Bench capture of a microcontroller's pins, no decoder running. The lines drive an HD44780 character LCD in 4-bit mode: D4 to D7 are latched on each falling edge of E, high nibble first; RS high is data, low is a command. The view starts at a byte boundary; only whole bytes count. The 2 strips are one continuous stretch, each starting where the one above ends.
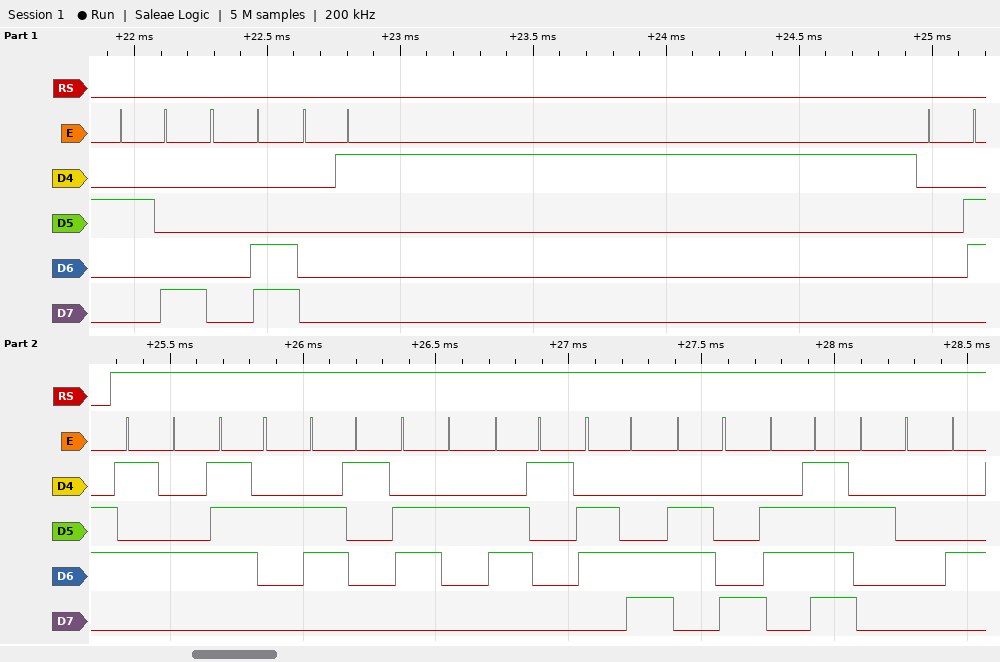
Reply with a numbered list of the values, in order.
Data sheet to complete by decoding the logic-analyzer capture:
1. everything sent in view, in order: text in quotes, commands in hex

1. 0x28 0x0C 0x01 0x06 "Trabalho "
